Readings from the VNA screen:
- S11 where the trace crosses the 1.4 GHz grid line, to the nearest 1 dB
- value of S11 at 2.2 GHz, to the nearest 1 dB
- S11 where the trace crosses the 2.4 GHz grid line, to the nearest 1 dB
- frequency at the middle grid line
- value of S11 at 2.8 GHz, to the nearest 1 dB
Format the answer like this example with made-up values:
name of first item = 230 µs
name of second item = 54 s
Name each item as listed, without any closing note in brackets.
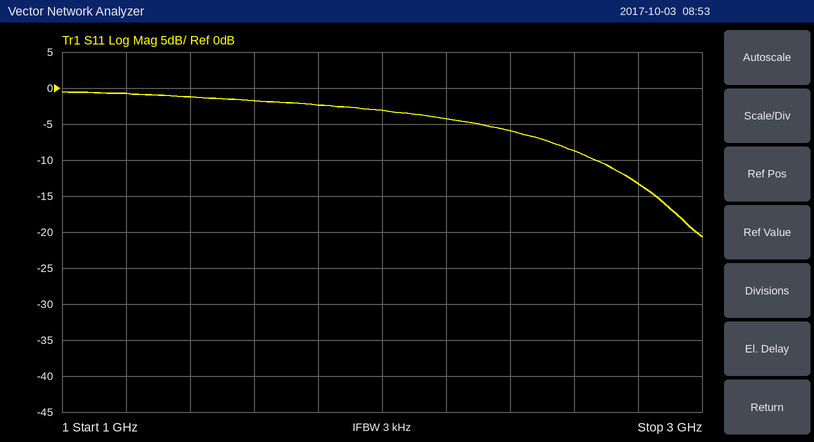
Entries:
S11 where the trace crosses the 1.4 GHz grid line, to the nearest 1 dB = -1 dB
value of S11 at 2.2 GHz, to the nearest 1 dB = -4 dB
S11 where the trace crosses the 2.4 GHz grid line, to the nearest 1 dB = -6 dB
frequency at the middle grid line = 2 GHz
value of S11 at 2.8 GHz, to the nearest 1 dB = -13 dB
